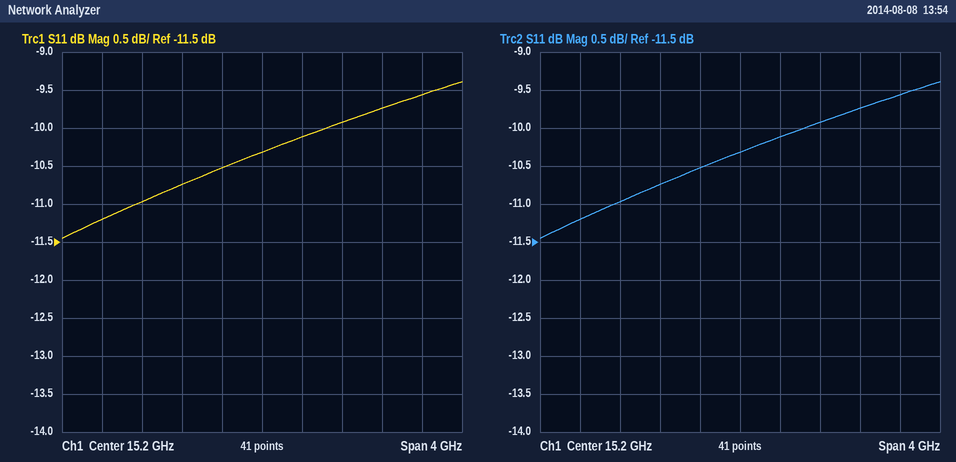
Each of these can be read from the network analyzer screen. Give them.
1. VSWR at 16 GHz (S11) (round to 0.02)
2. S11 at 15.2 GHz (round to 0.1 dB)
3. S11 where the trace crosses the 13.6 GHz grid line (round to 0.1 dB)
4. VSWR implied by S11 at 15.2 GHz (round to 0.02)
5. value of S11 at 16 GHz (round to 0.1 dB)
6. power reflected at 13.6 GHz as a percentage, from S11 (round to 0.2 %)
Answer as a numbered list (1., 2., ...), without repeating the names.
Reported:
1. 1.94
2. -10.3 dB
3. -11.2 dB
4. 1.88
5. -9.9 dB
6. 7.6 %
